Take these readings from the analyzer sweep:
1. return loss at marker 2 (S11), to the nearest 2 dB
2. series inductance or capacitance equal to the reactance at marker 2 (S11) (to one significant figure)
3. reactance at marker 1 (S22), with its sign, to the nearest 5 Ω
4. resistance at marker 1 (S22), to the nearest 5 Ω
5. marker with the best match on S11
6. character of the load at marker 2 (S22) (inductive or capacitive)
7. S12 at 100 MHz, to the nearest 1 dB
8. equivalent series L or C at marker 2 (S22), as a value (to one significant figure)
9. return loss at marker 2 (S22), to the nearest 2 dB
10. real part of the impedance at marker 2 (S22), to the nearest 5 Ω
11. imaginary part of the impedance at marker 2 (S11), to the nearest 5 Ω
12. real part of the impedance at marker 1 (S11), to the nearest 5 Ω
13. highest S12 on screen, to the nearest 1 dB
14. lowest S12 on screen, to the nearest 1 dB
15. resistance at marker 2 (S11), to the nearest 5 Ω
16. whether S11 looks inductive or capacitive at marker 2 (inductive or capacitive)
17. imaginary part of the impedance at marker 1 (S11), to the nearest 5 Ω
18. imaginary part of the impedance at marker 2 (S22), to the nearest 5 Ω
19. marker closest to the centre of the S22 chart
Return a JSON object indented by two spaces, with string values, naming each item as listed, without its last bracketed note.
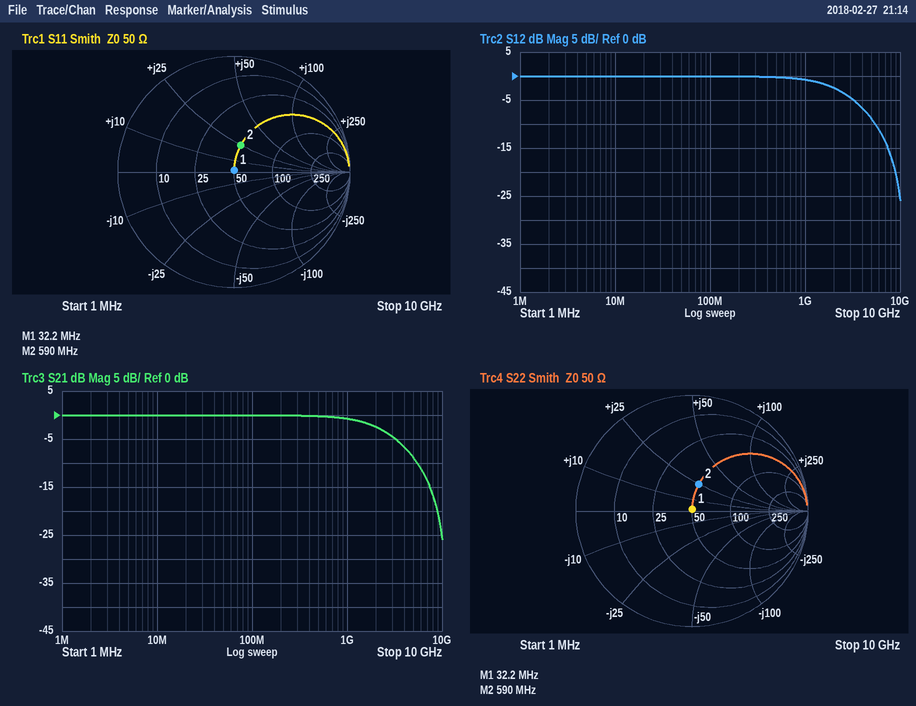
{
  "return loss at marker 2 (S11), to the nearest 2 dB": "12 dB",
  "series inductance or capacitance equal to the reactance at marker 2 (S11)": "7 nH",
  "reactance at marker 1 (S22), with its sign, to the nearest 5 Ω": "0 Ω",
  "resistance at marker 1 (S22), to the nearest 5 Ω": "50 Ω",
  "marker with the best match on S11": "marker 1",
  "character of the load at marker 2 (S22)": "inductive",
  "S12 at 100 MHz, to the nearest 1 dB": "0 dB",
  "equivalent series L or C at marker 2 (S22), as a value": "7 nH",
  "return loss at marker 2 (S22), to the nearest 2 dB": "12 dB",
  "real part of the impedance at marker 2 (S22), to the nearest 5 Ω": "50 Ω",
  "imaginary part of the impedance at marker 2 (S11), to the nearest 5 Ω": "+25 Ω",
  "real part of the impedance at marker 1 (S11), to the nearest 5 Ω": "50 Ω",
  "highest S12 on screen, to the nearest 1 dB": "0 dB",
  "lowest S12 on screen, to the nearest 1 dB": "-26 dB",
  "resistance at marker 2 (S11), to the nearest 5 Ω": "50 Ω",
  "whether S11 looks inductive or capacitive at marker 2": "inductive",
  "imaginary part of the impedance at marker 1 (S11), to the nearest 5 Ω": "0 Ω",
  "imaginary part of the impedance at marker 2 (S22), to the nearest 5 Ω": "+25 Ω",
  "marker closest to the centre of the S22 chart": "marker 1"
}
